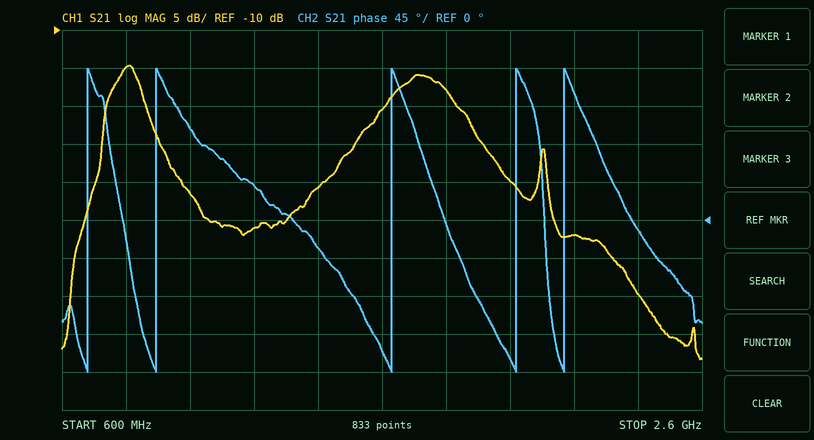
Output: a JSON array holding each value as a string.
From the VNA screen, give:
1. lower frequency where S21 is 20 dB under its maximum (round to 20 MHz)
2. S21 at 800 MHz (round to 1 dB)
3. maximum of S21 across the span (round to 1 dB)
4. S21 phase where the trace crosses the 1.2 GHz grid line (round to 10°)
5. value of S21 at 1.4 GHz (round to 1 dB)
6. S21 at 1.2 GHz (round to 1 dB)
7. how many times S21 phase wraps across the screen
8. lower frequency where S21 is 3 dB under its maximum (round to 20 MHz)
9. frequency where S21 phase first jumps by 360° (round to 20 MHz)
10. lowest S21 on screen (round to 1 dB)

["680 MHz", "-15 dB", "-15 dB", "40°", "-31 dB", "-36 dB", "5", "760 MHz", "680 MHz", "-53 dB"]
